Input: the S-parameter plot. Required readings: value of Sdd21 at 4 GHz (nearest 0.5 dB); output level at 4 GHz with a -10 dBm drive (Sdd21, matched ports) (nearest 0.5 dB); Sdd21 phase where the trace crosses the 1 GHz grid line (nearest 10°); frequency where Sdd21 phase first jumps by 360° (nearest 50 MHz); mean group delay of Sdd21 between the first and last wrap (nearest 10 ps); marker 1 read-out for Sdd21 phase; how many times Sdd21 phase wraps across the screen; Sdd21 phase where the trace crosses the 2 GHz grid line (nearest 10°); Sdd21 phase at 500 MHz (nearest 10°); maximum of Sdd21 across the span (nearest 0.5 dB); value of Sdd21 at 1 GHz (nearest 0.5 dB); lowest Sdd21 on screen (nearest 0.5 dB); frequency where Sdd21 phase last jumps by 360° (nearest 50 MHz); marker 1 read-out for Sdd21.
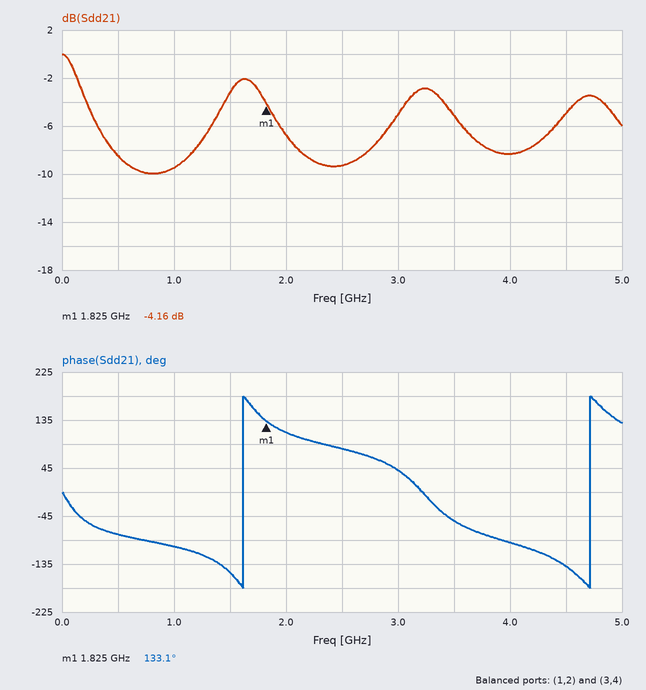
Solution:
-8.5 dB
-18.5 dBm
-100°
1.60 GHz
320 ps
133.1°
2
110°
-80°
0.0 dB
-9.5 dB
-10.0 dB
4.70 GHz
-4.16 dB
